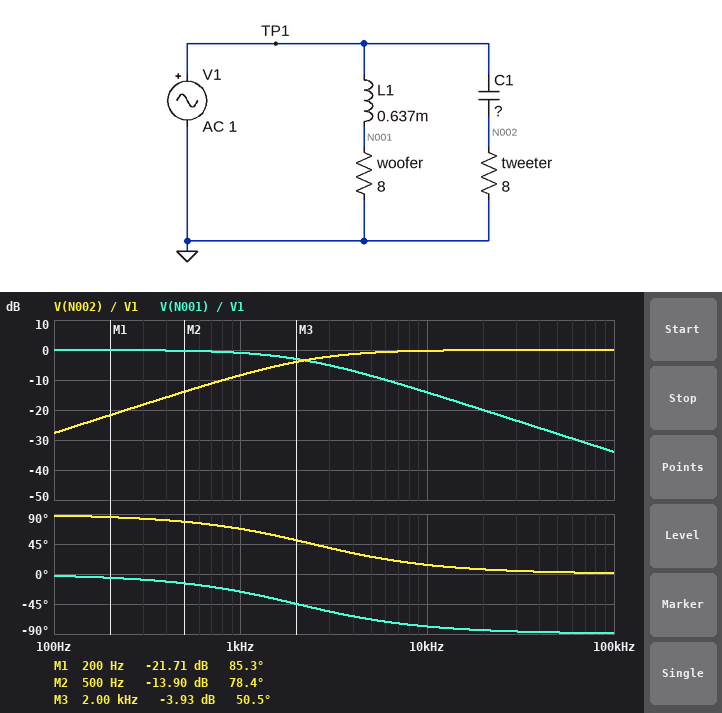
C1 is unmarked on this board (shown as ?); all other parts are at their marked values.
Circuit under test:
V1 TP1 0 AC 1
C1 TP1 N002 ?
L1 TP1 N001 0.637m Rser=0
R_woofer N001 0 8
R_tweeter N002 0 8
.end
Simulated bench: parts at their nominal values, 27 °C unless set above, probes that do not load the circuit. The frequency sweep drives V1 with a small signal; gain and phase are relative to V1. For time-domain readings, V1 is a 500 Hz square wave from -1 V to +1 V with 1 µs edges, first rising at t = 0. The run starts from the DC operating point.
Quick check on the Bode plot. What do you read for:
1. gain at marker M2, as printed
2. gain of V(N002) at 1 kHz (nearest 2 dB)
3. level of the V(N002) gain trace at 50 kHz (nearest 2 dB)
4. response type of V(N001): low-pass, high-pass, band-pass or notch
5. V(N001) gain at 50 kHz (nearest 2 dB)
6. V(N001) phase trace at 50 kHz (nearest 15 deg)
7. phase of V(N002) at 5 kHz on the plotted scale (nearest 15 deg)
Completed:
-13.90 dB
-8 dB
0 dB
low-pass
-28 dB
-90 deg
30 deg
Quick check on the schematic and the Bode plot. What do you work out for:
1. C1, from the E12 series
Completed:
8.2 µF
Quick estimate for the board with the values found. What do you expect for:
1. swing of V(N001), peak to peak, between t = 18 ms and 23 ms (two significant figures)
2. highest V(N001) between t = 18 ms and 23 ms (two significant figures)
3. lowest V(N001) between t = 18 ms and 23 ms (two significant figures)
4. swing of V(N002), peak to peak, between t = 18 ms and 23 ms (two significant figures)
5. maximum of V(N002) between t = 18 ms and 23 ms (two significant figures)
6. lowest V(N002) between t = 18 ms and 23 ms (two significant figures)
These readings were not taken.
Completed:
2.0 V
1.0 V
-1.0 V
4.0 V
2.0 V
-2.0 V
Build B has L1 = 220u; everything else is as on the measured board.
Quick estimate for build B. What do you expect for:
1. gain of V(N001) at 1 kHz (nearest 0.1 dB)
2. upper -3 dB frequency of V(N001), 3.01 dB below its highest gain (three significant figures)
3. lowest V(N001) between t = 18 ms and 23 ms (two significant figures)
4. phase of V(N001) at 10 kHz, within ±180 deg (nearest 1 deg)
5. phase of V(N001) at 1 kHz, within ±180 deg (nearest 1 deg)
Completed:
-0.1 dB
5.79 kHz
-1.0 V
-60 deg
-10 deg
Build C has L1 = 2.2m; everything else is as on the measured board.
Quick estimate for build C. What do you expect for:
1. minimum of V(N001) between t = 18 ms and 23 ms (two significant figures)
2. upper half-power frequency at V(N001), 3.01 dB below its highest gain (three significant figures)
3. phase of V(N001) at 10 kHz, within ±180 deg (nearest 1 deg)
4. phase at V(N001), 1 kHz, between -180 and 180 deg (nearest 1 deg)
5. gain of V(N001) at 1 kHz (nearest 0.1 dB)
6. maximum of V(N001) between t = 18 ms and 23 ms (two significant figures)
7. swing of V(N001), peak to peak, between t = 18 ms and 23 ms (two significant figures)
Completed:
-950 mV
579 Hz
-87 deg
-60 deg
-6.0 dB
950 mV
1.9 V
